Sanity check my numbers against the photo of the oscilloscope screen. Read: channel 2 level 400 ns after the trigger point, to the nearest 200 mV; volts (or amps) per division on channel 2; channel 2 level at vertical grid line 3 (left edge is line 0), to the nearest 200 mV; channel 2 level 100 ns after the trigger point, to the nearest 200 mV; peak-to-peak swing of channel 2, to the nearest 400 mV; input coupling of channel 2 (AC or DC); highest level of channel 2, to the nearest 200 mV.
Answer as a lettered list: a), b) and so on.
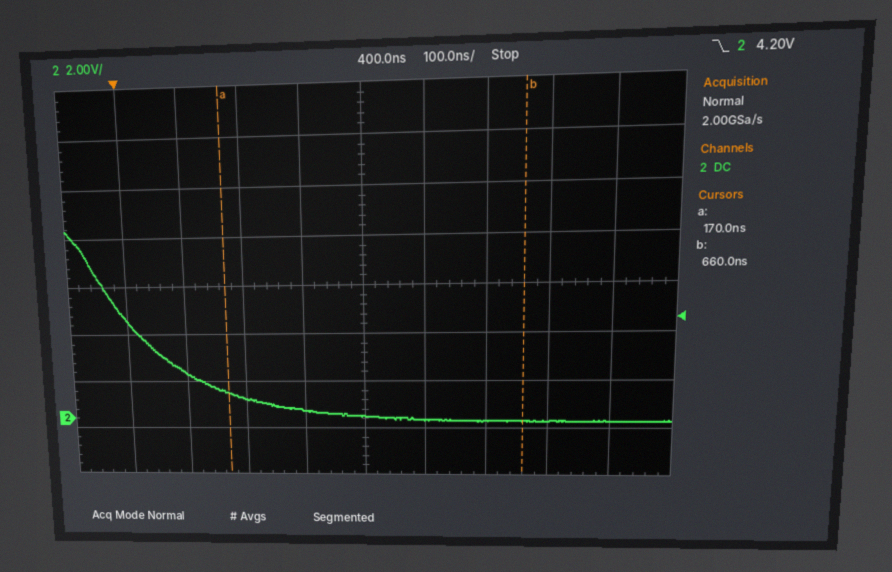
a) 200 mV
b) 2 V
c) 800 mV
d) 2.0 V
e) 8.0 V
f) DC
g) 8.0 V
